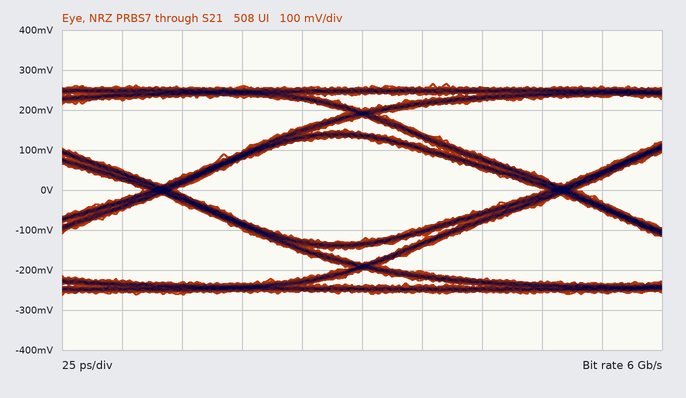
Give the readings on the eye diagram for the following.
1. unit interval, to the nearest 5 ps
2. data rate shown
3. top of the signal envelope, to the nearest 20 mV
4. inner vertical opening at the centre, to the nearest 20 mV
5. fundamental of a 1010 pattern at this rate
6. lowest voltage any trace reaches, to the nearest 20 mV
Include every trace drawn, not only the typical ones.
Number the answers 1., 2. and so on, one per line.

1. 165 ps
2. 6 Gb/s
3. 260 mV
4. 260 mV
5. 3 GHz
6. -260 mV
